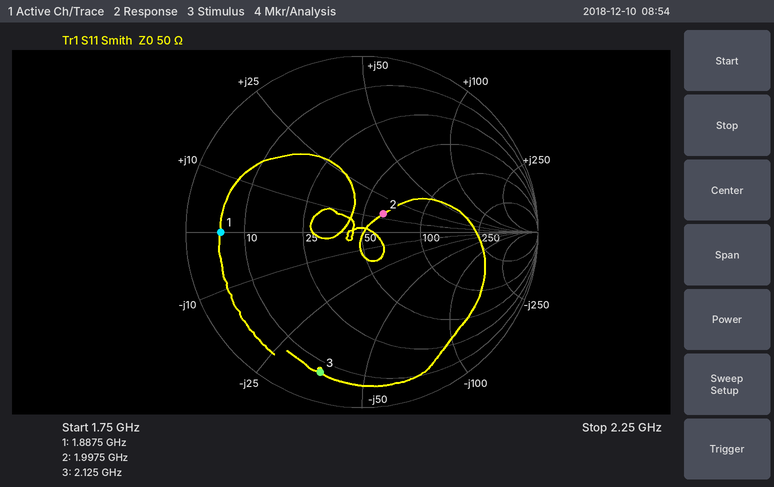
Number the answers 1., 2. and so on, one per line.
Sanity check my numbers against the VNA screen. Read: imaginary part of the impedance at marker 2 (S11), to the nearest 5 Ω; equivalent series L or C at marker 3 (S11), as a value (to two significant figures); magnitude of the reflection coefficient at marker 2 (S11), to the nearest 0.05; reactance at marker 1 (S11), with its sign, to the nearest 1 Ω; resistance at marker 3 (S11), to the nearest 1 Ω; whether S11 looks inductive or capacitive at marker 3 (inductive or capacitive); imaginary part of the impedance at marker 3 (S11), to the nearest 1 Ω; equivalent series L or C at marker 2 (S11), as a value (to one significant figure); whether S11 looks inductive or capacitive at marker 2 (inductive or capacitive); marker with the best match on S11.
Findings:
1. +15 Ω
2. 2.0 pF
3. 0.15
4. 0 Ω
5. 7 Ω
6. capacitive
7. -37 Ω
8. 1 nH
9. inductive
10. marker 2
